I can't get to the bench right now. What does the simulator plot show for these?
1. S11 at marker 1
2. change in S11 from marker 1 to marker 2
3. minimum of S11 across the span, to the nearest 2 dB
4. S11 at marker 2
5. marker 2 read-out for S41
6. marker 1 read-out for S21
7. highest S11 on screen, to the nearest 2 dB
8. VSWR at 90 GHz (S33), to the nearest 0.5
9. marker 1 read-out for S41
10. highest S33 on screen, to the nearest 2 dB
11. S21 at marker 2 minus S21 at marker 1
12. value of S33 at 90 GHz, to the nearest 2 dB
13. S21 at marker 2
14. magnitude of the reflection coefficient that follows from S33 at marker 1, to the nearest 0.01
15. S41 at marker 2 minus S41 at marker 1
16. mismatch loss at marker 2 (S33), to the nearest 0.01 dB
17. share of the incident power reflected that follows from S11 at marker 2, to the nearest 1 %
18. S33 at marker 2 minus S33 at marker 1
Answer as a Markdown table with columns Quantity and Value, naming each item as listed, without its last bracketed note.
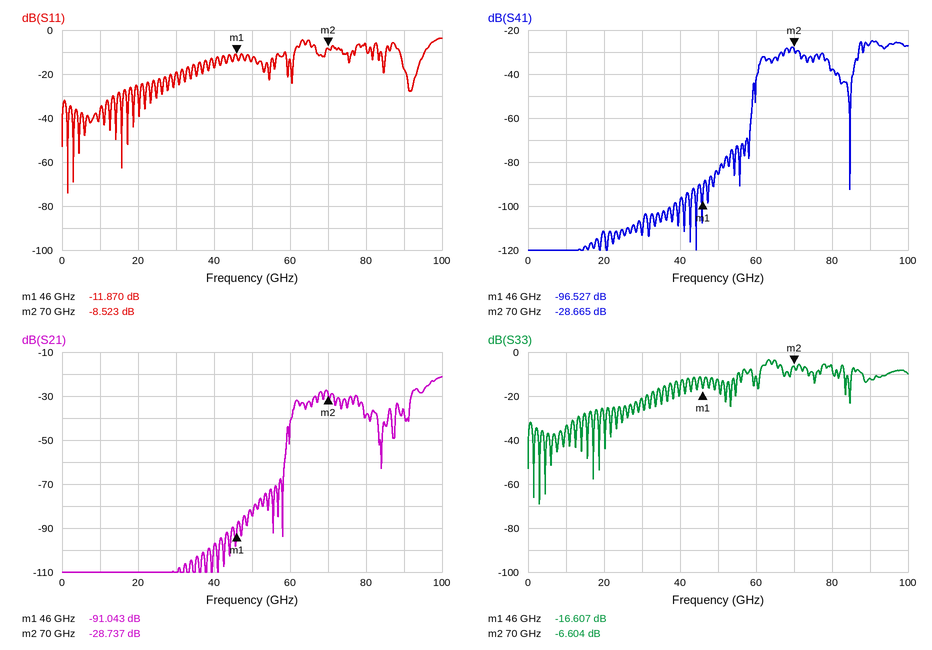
| Quantity | Value |
|---|---|
| S11 at marker 1 | -11.870 dB |
| change in S11 from marker 1 to marker 2 | 3.347 dB |
| minimum of S11 across the span, to the nearest 2 dB | -74 dB |
| S11 at marker 2 | -8.523 dB |
| marker 2 read-out for S41 | -28.665 dB |
| marker 1 read-out for S21 | -91.043 dB |
| highest S11 on screen, to the nearest 2 dB | -4 dB |
| VSWR at 90 GHz (S33), to the nearest 0.5 | 1.5 |
| marker 1 read-out for S41 | -96.527 dB |
| highest S33 on screen, to the nearest 2 dB | -4 dB |
| S21 at marker 2 minus S21 at marker 1 | 62.306 dB |
| value of S33 at 90 GHz, to the nearest 2 dB | -12 dB |
| S21 at marker 2 | -28.737 dB |
| magnitude of the reflection coefficient that follows from S33 at marker 1, to the nearest 0.01 | 0.15 |
| S41 at marker 2 minus S41 at marker 1 | 67.862 dB |
| mismatch loss at marker 2 (S33), to the nearest 0.01 dB | 1.07 dB |
| share of the incident power reflected that follows from S11 at marker 2, to the nearest 1 % | 14 % |
| S33 at marker 2 minus S33 at marker 1 | 10.003 dB |
